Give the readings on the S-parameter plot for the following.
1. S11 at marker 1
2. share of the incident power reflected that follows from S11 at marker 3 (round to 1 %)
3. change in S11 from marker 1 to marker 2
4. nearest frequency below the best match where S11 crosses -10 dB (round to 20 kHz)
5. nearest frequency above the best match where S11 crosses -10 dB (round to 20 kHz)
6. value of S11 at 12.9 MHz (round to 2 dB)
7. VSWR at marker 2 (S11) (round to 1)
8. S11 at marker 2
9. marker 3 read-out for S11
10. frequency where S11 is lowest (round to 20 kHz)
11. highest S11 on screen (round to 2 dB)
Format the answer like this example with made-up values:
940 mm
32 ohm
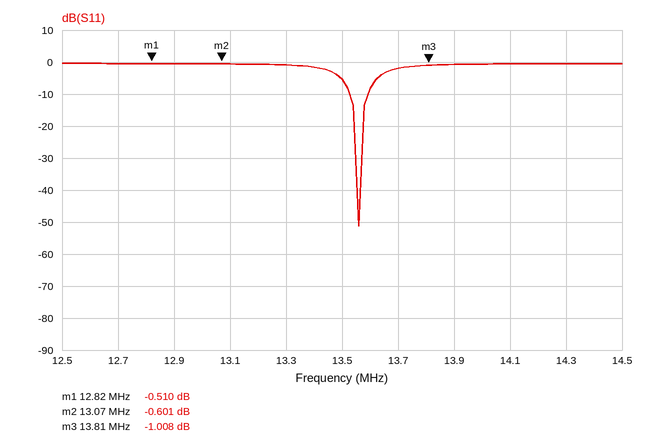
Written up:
-0.510 dB
79 %
-0.091 dB
13.52 MHz
13.60 MHz
0 dB
29
-0.601 dB
-1.008 dB
13.56 MHz
0 dB
